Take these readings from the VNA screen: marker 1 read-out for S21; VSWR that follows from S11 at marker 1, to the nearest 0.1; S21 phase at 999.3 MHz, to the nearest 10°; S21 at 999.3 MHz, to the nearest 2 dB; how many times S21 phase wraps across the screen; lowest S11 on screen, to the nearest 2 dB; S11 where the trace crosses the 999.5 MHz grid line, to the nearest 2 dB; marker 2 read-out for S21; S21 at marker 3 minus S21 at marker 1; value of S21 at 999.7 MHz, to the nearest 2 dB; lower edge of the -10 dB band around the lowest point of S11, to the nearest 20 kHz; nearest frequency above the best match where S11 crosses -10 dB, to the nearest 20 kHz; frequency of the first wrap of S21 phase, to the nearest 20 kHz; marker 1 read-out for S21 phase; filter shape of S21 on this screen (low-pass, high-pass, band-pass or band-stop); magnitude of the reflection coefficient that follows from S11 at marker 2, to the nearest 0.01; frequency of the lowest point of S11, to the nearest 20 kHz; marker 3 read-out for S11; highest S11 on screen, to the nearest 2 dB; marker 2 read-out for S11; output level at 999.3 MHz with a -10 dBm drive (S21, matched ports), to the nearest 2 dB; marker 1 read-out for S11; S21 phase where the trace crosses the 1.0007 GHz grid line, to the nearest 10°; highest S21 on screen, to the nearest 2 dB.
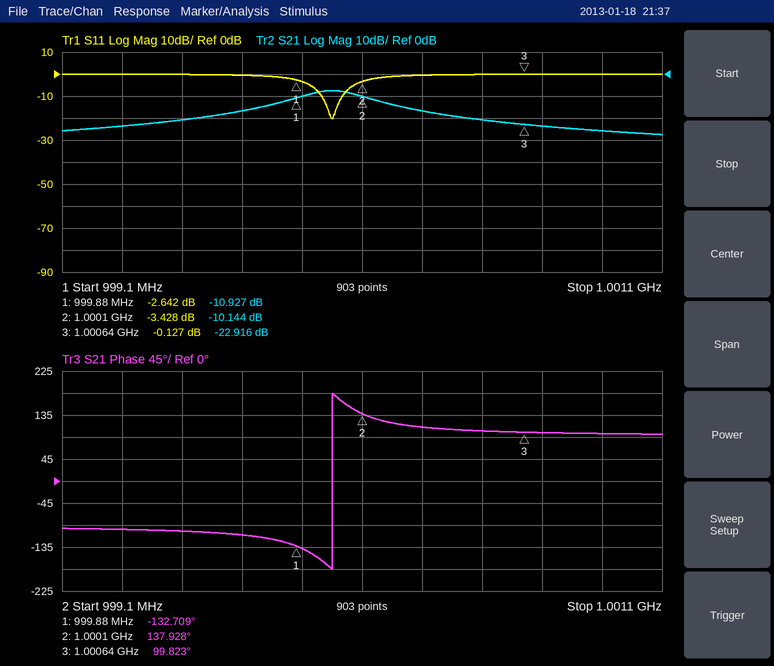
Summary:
-10.927 dB
6.6
-100°
-24 dB
1
-20 dB
0 dB
-10.144 dB
-11.989 dB
-16 dB
999.96 MHz
1.00004 GHz
1.00000 GHz
-132.709°
band-pass
0.67
1.00000 GHz
-0.127 dB
0 dB
-3.428 dB
-34 dBm
-2.642 dB
100°
-8 dB
